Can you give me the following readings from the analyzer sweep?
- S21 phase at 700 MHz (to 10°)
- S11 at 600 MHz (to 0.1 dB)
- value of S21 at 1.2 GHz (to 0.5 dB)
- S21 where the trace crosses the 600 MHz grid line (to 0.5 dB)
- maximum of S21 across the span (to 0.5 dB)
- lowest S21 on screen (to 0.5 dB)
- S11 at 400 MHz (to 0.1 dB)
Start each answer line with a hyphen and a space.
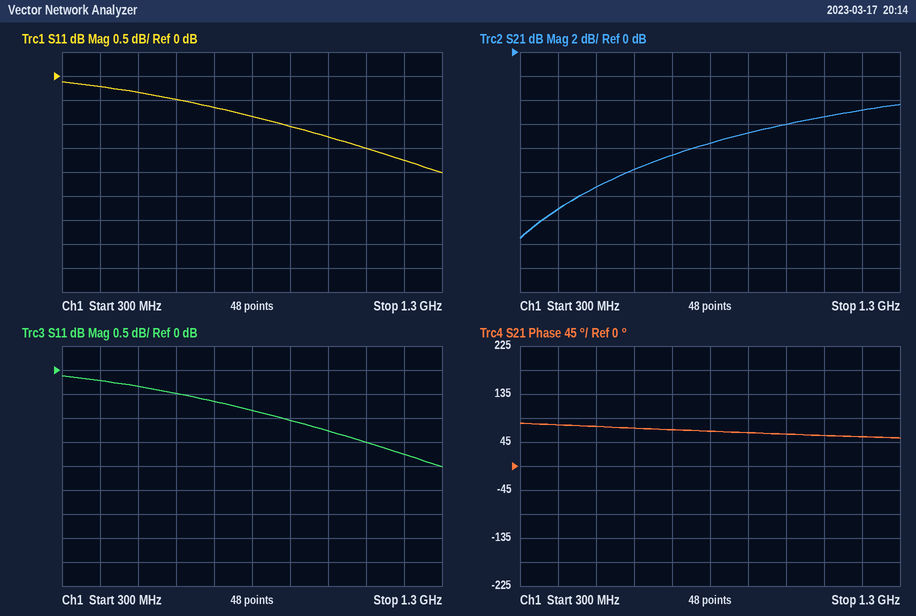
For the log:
- 70°
- -0.5 dB
- -5.0 dB
- -10.0 dB
- -4.5 dB
- -15.5 dB
- -0.2 dB
